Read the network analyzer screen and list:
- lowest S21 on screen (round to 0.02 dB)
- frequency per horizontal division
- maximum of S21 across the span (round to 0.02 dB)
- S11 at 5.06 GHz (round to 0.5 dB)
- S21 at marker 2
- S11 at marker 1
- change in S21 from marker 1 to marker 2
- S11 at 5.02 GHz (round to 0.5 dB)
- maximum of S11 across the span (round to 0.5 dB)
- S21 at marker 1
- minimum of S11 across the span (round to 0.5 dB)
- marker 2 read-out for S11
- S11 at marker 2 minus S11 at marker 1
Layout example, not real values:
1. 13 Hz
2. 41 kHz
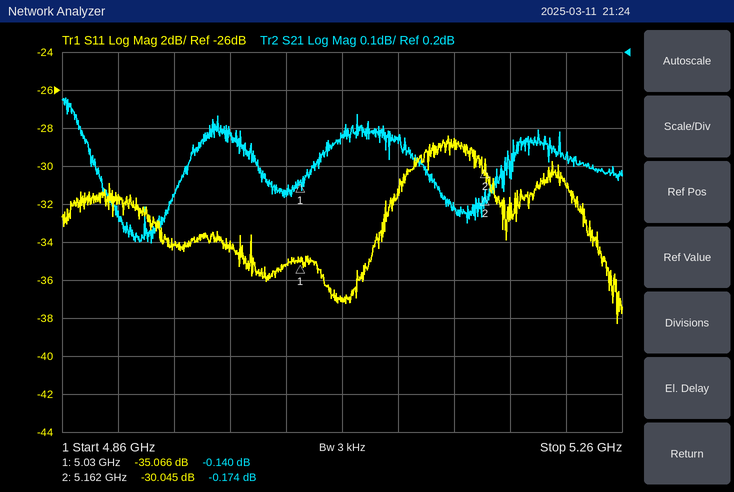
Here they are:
1. -0.30 dB
2. 40 MHz
3. 0.08 dB
4. -37.0 dB
5. -0.174 dB
6. -35.066 dB
7. -0.034 dB
8. -35.0 dB
9. -28.5 dB
10. -0.140 dB
11. -38.5 dB
12. -30.045 dB
13. 5.021 dB
